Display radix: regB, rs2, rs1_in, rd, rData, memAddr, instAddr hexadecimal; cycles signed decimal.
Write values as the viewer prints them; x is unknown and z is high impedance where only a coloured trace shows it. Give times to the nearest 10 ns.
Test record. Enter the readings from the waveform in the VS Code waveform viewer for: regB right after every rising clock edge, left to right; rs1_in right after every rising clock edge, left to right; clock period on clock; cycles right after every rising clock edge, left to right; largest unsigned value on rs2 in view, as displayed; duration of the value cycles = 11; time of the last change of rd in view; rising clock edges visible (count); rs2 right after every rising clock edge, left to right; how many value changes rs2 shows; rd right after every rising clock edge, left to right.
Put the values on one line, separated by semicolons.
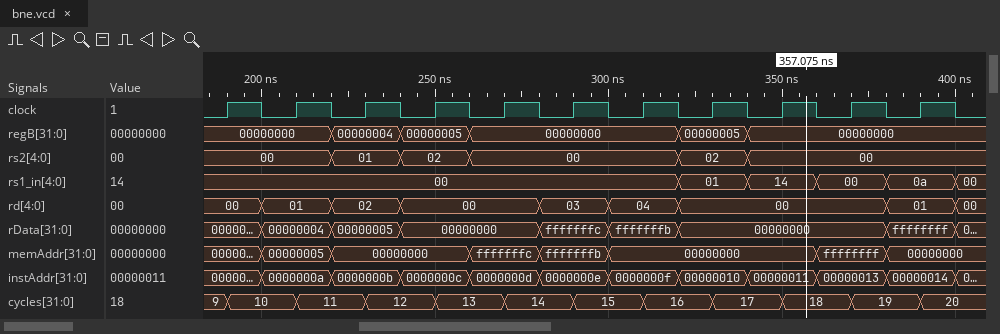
00000000, 00000000, 00000004, 00000005, 00000000, 00000000, 00000000, 00000005, 00000000, 00000000, 00000000; 00, 00, 00, 00, 00, 00, 00, 01, 14, 00, 0a; 20 ns; 10, 11, 12, 13, 14, 15, 16, 17, 18, 19, 20; 02; 20 ns; 400 ns; 11; 00, 00, 01, 02, 00, 00, 00, 02, 00, 00, 00; 5; 00, 01, 02, 00, 00, 03, 04, 00, 00, 00, 01
